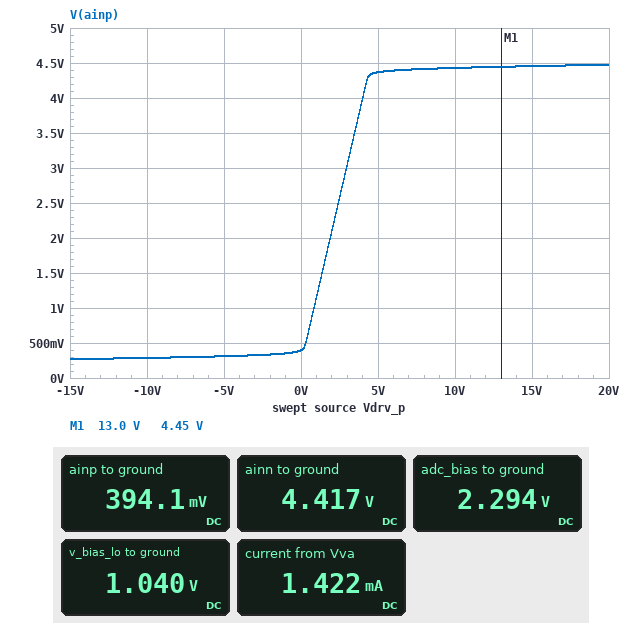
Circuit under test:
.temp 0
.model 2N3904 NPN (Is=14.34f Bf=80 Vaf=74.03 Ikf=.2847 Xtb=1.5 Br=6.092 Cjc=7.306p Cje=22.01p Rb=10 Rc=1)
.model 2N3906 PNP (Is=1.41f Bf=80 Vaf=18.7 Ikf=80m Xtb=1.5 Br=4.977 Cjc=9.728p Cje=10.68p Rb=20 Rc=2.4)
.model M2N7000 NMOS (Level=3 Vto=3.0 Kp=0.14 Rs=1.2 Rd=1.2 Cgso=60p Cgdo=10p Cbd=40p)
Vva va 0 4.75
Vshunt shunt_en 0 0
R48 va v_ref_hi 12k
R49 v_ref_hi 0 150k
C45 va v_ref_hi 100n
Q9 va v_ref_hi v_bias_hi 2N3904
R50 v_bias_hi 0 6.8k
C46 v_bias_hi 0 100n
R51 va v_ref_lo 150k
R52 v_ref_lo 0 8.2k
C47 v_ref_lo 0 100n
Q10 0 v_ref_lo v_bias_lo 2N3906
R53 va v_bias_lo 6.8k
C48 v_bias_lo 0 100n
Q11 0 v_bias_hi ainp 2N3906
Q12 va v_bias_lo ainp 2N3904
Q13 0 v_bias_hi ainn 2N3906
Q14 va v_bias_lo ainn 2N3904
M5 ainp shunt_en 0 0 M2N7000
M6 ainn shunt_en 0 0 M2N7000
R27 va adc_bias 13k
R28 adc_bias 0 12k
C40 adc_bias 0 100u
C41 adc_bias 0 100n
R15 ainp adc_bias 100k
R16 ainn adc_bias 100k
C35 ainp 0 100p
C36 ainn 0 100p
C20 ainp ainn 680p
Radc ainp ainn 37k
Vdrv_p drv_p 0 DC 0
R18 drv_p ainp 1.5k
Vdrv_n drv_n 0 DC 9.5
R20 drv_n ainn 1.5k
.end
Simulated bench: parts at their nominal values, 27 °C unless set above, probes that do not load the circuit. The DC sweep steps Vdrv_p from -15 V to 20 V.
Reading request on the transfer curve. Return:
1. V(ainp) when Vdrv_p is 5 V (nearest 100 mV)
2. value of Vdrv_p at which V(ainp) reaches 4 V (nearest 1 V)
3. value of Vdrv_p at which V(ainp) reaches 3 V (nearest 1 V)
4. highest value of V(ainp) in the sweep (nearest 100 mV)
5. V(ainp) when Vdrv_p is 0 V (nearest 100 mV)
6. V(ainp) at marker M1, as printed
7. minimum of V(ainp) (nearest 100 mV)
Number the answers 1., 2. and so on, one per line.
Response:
1. 4.4 V
2. 4 V
3. 3 V
4. 4.5 V
5. 400 mV
6. 4.45 V
7. 300 mV
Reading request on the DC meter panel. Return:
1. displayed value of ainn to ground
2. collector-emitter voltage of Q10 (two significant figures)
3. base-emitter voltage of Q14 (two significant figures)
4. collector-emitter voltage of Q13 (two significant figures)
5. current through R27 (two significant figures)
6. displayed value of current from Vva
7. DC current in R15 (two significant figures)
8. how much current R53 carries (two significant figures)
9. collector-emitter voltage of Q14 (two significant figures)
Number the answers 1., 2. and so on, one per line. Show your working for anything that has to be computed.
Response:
1. 4.417 V
2. 0 V - 1.04 V = -1.0 V
3. 1.04 V - 4.417 V = -3.4 V
4. 0 V - 4.417 V = -4.4 V
5. (4.75 V - 2.294 V) / 13 kΩ = 190 µA
6. 1.422 mA
7. (2.294 V - 394.1 mV) / 100 kΩ = 19 µA
8. (4.75 V - 1.04 V) / 6.8 kΩ = 550 µA
9. 4.75 V - 4.417 V = 330 mV
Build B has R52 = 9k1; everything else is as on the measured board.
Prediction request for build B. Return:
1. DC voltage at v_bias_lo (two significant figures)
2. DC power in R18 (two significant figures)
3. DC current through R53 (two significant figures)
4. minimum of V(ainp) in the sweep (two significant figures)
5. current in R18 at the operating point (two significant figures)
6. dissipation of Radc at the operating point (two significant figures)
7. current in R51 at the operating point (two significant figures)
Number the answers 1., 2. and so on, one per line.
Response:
1. 1.1 V
2. 120 µW
3. 540 µA
4. 300 mV
5. 280 µA
6. 430 µW
7. 29 µA
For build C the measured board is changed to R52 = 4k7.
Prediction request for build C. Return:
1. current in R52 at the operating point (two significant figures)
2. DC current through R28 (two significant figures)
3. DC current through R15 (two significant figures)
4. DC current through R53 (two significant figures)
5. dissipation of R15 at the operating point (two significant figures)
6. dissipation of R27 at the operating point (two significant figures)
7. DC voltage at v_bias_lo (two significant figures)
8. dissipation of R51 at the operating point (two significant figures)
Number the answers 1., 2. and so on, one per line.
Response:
1. 38 µA
2. 190 µA
3. 20 µA
4. 560 µA
5. 40 µW
6. 470 µW
7. 920 mV
8. 140 µW
